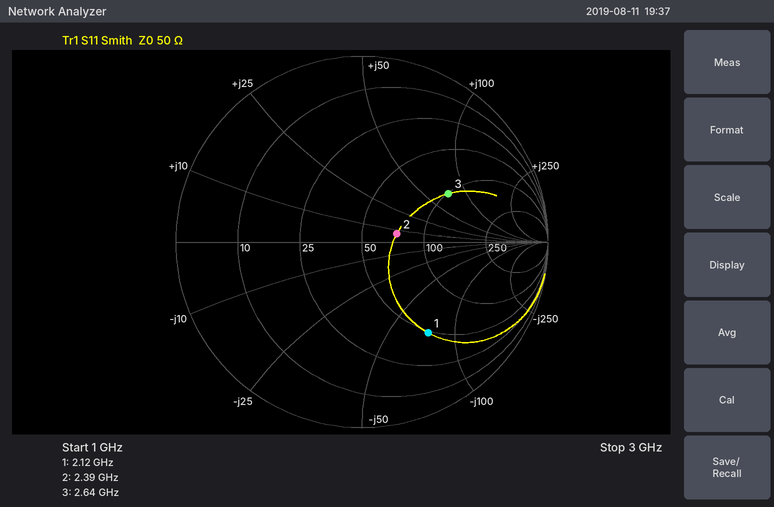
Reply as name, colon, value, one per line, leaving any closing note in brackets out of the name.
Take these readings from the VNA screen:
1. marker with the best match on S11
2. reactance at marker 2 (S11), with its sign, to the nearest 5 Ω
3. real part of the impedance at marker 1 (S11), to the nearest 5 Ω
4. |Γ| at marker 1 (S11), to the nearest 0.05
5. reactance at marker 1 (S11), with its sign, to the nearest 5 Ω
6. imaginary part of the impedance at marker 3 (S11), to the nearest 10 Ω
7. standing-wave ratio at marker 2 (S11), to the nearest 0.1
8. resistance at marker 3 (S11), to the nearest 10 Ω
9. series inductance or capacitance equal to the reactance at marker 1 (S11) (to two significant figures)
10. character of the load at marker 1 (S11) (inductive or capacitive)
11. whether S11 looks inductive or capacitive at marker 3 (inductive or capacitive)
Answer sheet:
marker with the best match on S11: marker 2
reactance at marker 2 (S11), with its sign, to the nearest 5 Ω: +5 Ω
real part of the impedance at marker 1 (S11), to the nearest 5 Ω: 50 Ω
|Γ| at marker 1 (S11), to the nearest 0.05: 0.60
reactance at marker 1 (S11), with its sign, to the nearest 5 Ω: -75 Ω
imaginary part of the impedance at marker 3 (S11), to the nearest 10 Ω: +70 Ω
standing-wave ratio at marker 2 (S11), to the nearest 0.1: 1.5
resistance at marker 3 (S11), to the nearest 10 Ω: 100 Ω
series inductance or capacitance equal to the reactance at marker 1 (S11): 1.0 pF
character of the load at marker 1 (S11): capacitive
whether S11 looks inductive or capacitive at marker 3: inductive
